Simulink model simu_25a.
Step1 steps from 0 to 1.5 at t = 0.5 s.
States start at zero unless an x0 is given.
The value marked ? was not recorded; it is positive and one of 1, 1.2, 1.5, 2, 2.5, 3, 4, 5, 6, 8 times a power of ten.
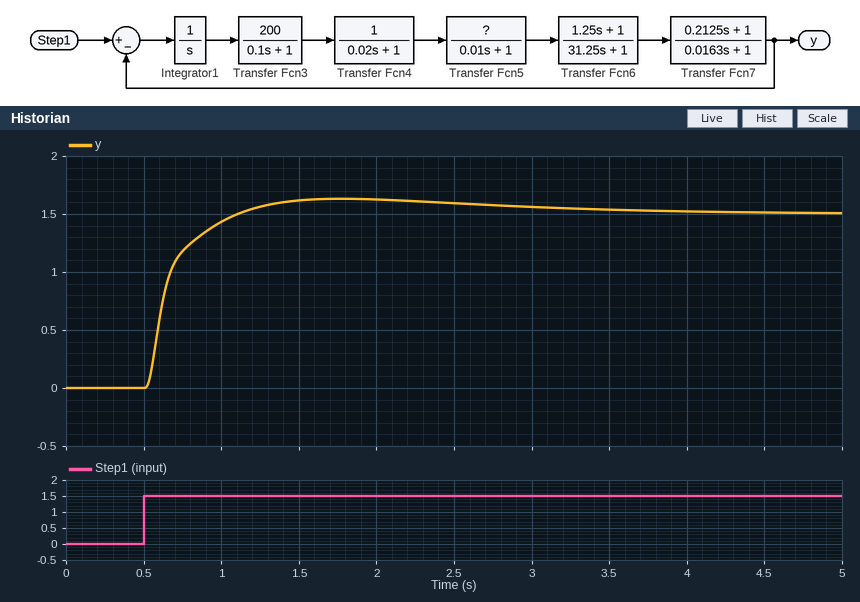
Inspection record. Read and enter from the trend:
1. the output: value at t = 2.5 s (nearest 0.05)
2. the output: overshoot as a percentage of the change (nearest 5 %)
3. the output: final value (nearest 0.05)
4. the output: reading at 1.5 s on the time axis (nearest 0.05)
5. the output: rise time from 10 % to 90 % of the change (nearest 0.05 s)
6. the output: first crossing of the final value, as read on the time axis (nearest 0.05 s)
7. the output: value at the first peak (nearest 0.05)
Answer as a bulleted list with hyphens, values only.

- 1.60
- 10 %
- 1.50
- 1.60
- 0.35 s
- 1.10 s
- 1.65
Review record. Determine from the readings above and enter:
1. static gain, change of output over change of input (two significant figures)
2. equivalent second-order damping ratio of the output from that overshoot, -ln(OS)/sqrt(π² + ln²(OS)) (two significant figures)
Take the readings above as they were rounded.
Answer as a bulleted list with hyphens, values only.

- 1.0
- 0.59
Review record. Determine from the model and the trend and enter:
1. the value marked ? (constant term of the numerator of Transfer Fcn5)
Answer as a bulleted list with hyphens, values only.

- 0.5
